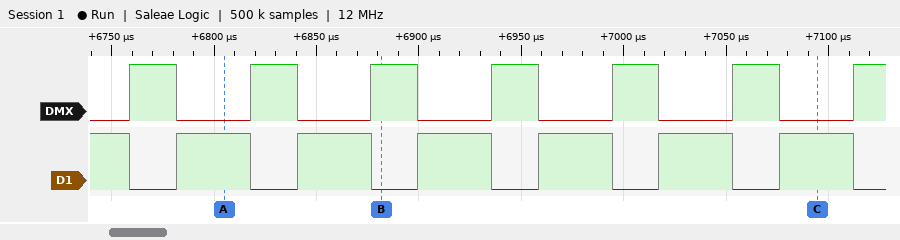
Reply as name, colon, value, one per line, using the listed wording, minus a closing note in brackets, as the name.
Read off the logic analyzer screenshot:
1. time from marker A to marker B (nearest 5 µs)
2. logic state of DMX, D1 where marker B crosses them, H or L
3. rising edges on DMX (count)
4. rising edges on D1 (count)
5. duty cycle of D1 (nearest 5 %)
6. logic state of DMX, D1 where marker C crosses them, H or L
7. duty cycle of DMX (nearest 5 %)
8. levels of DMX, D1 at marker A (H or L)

time from marker A to marker B: 75 µs
logic state of DMX, D1 where marker B crosses them, H or L: DMX=H, D1=L
rising edges on DMX: 7
rising edges on D1: 6
duty cycle of D1: 60 %
logic state of DMX, D1 where marker C crosses them, H or L: DMX=L, D1=H
duty cycle of DMX: 40 %
levels of DMX, D1 at marker A: DMX=L, D1=H
